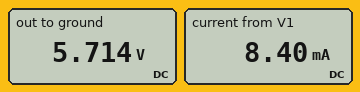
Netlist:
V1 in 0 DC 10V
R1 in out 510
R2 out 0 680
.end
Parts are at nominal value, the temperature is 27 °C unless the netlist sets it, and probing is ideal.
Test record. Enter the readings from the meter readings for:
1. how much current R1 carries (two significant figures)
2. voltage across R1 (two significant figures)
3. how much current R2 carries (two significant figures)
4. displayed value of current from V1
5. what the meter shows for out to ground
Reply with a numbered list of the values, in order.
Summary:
1. 8.4 mA
2. 4.3 V
3. 8.4 mA
4. 8.40 mA
5. 5.714 V
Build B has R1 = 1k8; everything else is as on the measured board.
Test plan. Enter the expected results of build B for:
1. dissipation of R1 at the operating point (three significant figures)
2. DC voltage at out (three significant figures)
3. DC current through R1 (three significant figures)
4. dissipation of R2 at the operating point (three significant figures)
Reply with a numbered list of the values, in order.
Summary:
1. 29.3 mW
2. 2.74 V
3. 4.03 mA
4. 11.1 mW
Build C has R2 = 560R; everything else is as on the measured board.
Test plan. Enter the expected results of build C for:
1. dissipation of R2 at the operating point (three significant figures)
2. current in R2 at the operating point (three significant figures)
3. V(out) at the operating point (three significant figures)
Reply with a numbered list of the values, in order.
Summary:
1. 48.9 mW
2. 9.35 mA
3. 5.23 V
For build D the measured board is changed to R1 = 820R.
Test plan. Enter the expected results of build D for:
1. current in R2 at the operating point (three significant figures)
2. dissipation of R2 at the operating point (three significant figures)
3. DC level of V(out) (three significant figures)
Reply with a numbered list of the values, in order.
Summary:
1. 6.67 mA
2. 30.2 mW
3. 4.53 V
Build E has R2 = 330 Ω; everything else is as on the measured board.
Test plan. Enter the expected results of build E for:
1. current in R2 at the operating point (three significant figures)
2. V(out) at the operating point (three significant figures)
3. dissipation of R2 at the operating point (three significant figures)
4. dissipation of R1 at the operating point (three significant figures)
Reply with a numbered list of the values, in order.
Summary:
1. 11.9 mA
2. 3.93 V
3. 46.8 mW
4. 72.3 mW
